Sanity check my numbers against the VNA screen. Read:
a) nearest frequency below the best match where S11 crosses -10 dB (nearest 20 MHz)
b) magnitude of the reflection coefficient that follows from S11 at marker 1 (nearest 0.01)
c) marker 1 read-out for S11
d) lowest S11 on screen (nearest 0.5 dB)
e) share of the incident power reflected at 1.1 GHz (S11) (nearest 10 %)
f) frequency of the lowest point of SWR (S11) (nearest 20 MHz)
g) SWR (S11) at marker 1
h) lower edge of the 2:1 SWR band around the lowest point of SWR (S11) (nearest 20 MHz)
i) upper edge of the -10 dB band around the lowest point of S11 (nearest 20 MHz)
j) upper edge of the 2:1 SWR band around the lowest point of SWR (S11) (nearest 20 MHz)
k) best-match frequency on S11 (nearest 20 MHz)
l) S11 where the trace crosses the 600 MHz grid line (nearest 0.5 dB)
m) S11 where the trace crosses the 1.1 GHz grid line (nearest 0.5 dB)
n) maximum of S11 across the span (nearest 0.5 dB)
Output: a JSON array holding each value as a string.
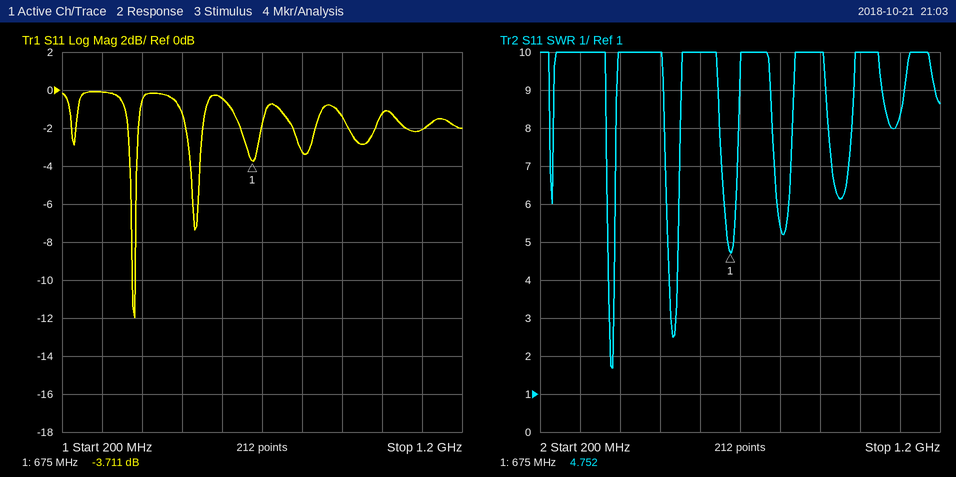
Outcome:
["380 MHz", "0.65", "-3.711 dB", "-12.0 dB", "60 %", "380 MHz", "4.752", "380 MHz", "380 MHz", "380 MHz", "380 MHz", "-0.5 dB", "-2.0 dB", "0.0 dB"]
